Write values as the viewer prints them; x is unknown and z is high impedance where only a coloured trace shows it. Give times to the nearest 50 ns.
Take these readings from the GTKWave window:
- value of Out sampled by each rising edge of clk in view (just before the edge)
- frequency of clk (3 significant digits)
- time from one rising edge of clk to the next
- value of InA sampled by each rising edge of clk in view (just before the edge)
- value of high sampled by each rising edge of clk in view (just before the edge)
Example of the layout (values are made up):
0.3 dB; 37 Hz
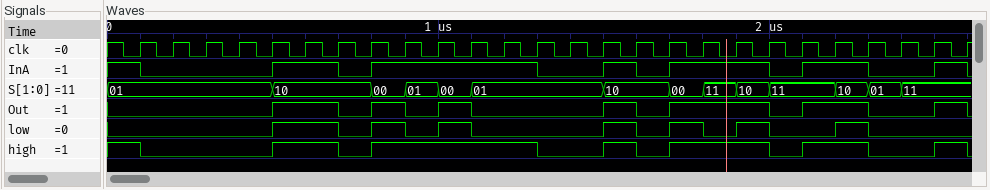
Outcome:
0 0 0 0 0 1 1 0 1 0 1 0 0 0 0 1 0 1 1 1 0 1 1 0 0 1; 10.0 MHz; 100 ns; 1 0 0 0 0 1 1 0 1 1 1 1 1 0 0 1 0 1 1 1 0 1 1 0 0 1; 1 0 0 0 0 1 1 0 1 1 1 1 1 0 0 1 0 1 1 1 0 1 1 0 0 1
